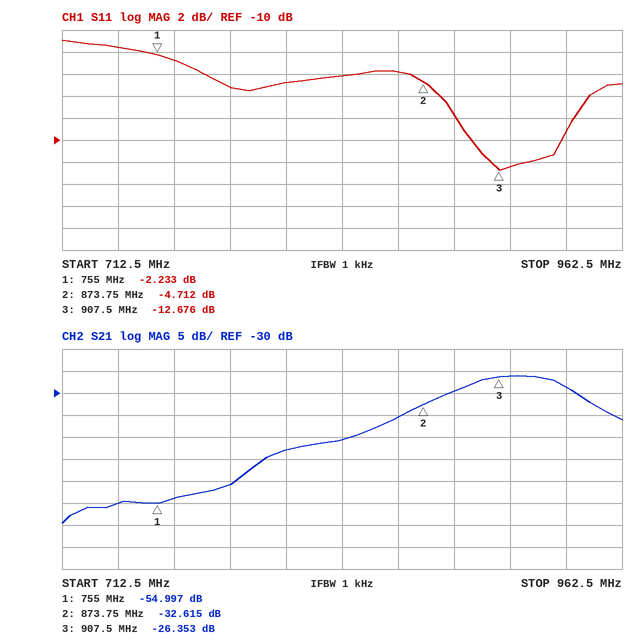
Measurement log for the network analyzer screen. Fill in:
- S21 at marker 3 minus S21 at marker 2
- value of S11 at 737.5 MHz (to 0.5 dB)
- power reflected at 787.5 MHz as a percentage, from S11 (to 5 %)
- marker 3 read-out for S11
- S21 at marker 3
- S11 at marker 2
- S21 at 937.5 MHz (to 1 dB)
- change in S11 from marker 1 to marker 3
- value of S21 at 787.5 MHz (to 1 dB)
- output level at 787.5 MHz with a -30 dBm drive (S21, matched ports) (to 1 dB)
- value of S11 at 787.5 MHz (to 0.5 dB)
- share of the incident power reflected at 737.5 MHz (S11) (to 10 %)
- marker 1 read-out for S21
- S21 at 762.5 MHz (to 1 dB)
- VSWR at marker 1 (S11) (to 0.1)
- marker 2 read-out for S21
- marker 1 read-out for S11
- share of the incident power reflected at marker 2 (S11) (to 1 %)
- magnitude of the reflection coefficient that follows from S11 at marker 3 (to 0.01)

6.262 dB
-1.5 dB
30 %
-12.676 dB
-26.353 dB
-4.712 dB
-29 dB
-10.443 dB
-51 dB
-81 dBm
-5.0 dB
70 %
-54.997 dB
-54 dB
7.8
-32.615 dB
-2.233 dB
34 %
0.23
